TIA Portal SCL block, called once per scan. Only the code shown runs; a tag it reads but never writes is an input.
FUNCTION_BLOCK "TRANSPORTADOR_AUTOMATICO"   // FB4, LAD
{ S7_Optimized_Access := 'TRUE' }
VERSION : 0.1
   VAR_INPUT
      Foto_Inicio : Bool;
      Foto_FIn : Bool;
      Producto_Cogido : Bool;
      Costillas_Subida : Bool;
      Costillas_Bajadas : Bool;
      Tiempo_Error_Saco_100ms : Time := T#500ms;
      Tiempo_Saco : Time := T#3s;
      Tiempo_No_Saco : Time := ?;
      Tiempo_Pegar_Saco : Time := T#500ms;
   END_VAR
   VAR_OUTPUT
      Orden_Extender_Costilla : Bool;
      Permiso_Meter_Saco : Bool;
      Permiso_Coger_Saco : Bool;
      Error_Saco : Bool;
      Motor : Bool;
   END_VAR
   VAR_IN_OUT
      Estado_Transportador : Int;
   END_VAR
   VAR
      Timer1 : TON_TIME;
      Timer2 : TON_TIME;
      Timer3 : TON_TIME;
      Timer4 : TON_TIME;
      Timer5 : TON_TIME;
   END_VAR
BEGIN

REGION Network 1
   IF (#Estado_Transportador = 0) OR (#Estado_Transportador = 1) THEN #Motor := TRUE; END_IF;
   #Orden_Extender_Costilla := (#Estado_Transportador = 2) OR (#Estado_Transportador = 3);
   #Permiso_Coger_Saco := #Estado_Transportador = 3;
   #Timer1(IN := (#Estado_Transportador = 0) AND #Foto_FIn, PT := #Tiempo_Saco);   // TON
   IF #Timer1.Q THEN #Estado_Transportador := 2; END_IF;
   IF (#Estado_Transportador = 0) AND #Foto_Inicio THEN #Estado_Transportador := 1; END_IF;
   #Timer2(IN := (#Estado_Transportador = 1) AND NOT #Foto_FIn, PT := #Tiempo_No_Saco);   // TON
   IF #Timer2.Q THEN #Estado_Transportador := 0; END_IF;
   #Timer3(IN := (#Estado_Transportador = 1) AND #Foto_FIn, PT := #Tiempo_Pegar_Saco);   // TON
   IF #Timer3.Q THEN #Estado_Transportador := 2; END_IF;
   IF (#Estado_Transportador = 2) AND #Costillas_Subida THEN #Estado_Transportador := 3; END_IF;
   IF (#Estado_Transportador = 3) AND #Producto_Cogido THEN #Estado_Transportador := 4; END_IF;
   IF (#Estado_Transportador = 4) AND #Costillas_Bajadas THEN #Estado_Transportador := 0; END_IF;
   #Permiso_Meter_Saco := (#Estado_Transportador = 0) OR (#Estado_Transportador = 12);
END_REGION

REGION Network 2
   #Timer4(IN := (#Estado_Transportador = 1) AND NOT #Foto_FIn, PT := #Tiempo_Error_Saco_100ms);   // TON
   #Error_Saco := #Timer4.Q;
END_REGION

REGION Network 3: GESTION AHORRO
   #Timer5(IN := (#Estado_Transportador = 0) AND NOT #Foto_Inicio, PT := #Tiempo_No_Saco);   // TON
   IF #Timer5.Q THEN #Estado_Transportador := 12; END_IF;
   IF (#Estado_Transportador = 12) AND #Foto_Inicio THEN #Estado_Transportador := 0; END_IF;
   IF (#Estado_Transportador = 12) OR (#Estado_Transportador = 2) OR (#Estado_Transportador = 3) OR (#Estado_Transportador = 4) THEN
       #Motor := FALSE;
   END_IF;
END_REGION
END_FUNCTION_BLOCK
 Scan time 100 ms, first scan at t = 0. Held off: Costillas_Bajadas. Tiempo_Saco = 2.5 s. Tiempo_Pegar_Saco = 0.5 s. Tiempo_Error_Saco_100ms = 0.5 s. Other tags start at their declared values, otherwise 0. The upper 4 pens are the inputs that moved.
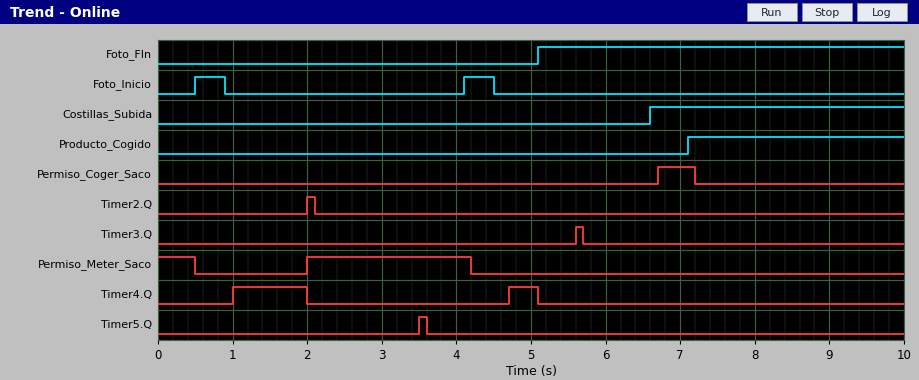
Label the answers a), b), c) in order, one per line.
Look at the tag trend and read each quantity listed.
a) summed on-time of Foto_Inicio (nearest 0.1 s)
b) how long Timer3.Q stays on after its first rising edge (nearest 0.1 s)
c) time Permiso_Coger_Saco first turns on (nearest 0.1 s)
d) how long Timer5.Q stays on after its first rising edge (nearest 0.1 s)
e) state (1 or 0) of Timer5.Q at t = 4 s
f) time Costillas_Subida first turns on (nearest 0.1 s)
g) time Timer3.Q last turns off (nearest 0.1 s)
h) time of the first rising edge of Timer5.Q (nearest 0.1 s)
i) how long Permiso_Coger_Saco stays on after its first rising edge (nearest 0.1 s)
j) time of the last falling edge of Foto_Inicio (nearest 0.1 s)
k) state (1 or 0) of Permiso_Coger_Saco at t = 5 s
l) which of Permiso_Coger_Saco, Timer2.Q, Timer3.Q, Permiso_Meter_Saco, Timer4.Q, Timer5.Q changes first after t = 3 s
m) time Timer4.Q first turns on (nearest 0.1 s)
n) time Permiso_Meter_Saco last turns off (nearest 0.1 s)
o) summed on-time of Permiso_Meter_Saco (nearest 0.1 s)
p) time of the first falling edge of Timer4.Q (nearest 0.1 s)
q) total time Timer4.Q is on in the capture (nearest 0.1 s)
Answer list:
a) 0.8 s
b) 0.1 s
c) 6.7 s
d) 0.1 s
e) 0
f) 6.6 s
g) 5.7 s
h) 3.5 s
i) 0.5 s
j) 4.5 s
k) 0
l) Timer5.Q
m) 1.0 s
n) 4.2 s
o) 2.7 s
p) 2.0 s
q) 1.4 s
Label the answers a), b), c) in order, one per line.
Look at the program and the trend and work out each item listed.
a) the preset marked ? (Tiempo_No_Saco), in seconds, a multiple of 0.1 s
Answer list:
a) 1.5 s
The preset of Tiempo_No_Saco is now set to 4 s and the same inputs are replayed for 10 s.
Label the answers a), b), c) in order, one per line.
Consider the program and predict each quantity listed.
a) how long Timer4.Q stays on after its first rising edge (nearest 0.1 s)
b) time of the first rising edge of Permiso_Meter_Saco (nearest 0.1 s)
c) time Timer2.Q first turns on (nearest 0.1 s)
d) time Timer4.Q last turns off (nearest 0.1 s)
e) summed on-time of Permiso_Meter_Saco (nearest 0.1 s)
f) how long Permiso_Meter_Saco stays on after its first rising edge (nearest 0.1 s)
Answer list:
a) 3.5 s
b) 4.5 s
c) 4.5 s
d) 4.5 s
e) 3.6 s
f) 3.1 s
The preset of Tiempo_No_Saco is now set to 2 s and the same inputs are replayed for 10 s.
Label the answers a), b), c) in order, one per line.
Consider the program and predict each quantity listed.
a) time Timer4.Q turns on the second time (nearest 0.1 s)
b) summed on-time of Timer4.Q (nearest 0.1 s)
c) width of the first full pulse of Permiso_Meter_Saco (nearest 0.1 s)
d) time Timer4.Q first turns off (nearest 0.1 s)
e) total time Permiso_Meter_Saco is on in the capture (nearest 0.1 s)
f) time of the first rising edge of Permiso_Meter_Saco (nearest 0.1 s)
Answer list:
a) 4.6 s
b) 2.0 s
c) 1.6 s
d) 2.5 s
e) 2.1 s
f) 2.5 s
